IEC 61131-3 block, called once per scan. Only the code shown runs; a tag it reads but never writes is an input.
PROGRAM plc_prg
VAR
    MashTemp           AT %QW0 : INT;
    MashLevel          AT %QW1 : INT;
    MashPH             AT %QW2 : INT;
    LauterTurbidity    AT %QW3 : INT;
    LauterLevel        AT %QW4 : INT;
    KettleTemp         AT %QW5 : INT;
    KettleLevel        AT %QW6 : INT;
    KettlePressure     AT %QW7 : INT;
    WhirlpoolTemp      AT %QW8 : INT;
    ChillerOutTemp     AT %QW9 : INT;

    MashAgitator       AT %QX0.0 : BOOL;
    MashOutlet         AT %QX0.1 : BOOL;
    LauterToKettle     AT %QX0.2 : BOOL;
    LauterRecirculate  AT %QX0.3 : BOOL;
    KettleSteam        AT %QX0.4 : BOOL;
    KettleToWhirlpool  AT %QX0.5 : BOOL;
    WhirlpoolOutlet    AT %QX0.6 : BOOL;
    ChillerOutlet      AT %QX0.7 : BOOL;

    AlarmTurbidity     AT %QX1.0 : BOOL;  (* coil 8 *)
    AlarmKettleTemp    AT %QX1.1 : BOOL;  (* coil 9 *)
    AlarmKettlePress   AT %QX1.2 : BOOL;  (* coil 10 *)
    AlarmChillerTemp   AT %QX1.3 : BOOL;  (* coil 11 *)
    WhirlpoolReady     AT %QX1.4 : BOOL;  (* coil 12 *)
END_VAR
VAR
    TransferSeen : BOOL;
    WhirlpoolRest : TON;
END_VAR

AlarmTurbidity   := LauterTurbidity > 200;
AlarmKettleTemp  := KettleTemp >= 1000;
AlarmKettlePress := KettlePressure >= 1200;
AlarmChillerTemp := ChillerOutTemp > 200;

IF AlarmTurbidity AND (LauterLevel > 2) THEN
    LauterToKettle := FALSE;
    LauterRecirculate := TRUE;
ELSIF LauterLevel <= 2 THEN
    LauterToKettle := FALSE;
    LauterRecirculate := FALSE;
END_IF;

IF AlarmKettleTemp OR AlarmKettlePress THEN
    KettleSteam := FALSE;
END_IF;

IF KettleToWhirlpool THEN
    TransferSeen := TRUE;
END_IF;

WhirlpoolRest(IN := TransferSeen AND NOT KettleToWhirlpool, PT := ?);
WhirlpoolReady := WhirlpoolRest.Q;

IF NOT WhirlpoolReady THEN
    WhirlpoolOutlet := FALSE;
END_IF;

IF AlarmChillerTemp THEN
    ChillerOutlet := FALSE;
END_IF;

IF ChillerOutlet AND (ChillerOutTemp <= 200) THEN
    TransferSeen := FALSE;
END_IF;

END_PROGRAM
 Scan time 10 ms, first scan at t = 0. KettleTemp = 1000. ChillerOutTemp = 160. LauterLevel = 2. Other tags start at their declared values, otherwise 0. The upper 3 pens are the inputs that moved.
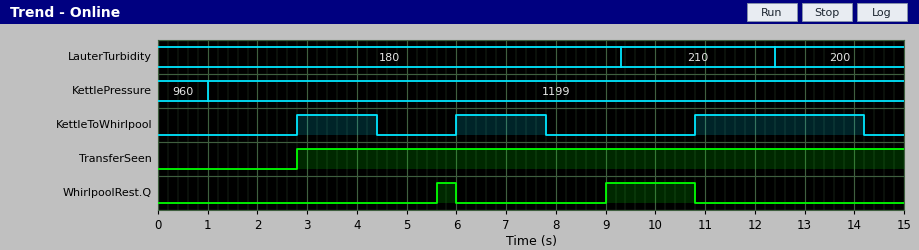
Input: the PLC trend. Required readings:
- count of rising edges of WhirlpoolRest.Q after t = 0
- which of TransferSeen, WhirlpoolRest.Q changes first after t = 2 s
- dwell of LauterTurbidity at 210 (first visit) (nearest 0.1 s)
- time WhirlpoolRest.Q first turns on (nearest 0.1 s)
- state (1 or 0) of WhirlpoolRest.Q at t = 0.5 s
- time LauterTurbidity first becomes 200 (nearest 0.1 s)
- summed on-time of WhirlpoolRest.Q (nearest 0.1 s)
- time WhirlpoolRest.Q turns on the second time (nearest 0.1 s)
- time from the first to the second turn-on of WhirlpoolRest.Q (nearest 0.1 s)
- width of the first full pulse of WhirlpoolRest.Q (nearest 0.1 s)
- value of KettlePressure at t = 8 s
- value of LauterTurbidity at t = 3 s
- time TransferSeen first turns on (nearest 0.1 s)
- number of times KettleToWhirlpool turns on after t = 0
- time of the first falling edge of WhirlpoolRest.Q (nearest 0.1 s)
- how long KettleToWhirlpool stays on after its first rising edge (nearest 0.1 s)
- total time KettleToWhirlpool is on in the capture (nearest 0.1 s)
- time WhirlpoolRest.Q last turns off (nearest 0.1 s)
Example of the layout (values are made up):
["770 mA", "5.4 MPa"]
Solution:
["2", "TransferSeen", "3.1 s", "5.6 s", "0", "12.4 s", "2.2 s", "9.0 s", "3.4 s", "0.4 s", "1199", "180", "2.8 s", "3", "6.0 s", "1.6 s", "6.8 s", "10.8 s"]
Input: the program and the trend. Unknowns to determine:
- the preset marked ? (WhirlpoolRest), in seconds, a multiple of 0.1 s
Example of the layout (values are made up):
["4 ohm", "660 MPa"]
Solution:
["1.2 s"]
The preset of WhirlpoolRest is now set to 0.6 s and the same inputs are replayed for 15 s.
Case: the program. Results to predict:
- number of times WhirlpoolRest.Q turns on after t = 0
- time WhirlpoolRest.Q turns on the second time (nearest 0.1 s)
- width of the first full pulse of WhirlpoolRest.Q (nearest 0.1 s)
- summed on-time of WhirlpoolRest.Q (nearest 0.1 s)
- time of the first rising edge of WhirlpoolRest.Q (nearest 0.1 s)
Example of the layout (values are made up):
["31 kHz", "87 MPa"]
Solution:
["3", "8.4 s", "1.0 s", "3.6 s", "5.0 s"]
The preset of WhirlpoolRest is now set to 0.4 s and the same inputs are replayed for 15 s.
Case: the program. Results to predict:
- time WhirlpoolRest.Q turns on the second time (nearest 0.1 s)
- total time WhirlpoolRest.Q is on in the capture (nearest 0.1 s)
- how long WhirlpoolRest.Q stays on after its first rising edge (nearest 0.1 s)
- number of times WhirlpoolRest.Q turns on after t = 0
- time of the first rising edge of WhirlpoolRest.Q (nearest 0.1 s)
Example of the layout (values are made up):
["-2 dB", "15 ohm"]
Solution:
["8.2 s", "4.2 s", "1.2 s", "3", "4.8 s"]
